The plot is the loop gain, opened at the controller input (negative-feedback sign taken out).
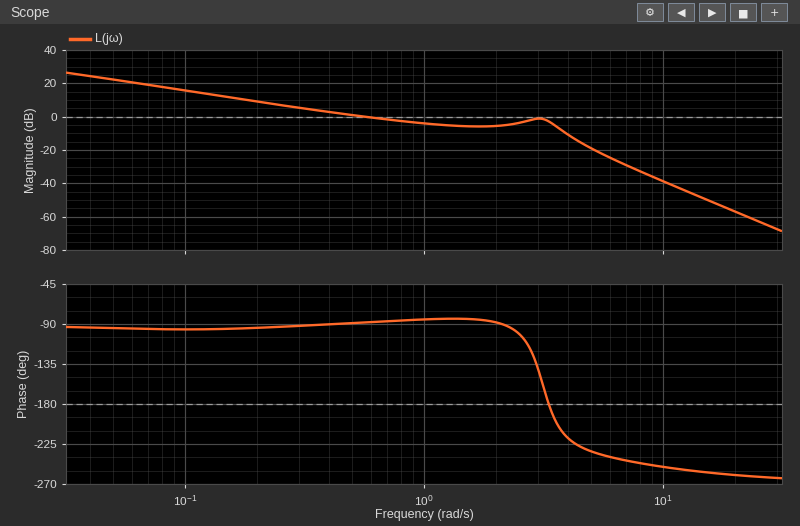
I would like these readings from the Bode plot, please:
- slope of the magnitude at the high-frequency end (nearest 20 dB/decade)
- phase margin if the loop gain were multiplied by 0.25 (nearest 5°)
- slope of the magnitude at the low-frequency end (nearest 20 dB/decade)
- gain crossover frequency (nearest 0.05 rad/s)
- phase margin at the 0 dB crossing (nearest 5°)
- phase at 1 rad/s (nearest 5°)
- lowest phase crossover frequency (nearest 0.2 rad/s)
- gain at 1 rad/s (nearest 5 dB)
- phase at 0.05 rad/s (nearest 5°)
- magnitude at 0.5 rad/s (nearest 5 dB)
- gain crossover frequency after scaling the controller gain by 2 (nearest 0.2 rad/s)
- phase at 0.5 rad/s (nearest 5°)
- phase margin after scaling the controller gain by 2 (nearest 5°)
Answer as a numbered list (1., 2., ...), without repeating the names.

1. -60 dB/decade
2. 85°
3. -20 dB/decade
4. 0.55 rad/s
5. 90°
6. -85°
7. 3.4 rad/s
8. -5 dB
9. -95°
10. 0 dB
11. 3.6 rad/s
12. -90°
13. -20°
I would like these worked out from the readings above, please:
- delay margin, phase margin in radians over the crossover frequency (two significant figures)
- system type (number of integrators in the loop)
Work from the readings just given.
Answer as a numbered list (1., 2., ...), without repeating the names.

1. 2.9 s
2. 1
